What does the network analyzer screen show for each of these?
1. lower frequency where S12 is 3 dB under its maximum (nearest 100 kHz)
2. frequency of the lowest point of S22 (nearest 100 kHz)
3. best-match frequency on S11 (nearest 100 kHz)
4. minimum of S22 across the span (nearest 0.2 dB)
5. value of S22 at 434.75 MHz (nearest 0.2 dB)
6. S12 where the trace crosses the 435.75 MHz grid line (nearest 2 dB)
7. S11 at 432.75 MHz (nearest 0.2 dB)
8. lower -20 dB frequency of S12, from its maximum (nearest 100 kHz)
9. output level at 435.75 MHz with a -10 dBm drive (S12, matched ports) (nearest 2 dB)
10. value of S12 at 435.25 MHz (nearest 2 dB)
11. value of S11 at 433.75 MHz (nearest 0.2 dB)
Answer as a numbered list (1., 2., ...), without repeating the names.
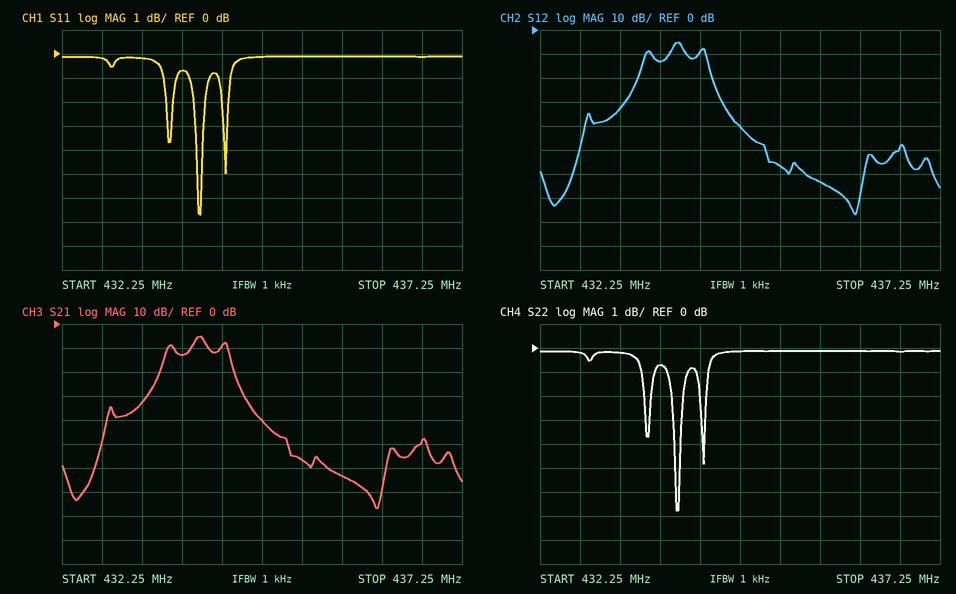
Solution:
1. 433.9 MHz
2. 434.0 MHz
3. 434.0 MHz
4. -6.8 dB
5. -0.2 dB
6. -64 dB
7. -0.2 dB
8. 433.4 MHz
9. -74 dBm
10. -56 dB
11. -0.6 dB
